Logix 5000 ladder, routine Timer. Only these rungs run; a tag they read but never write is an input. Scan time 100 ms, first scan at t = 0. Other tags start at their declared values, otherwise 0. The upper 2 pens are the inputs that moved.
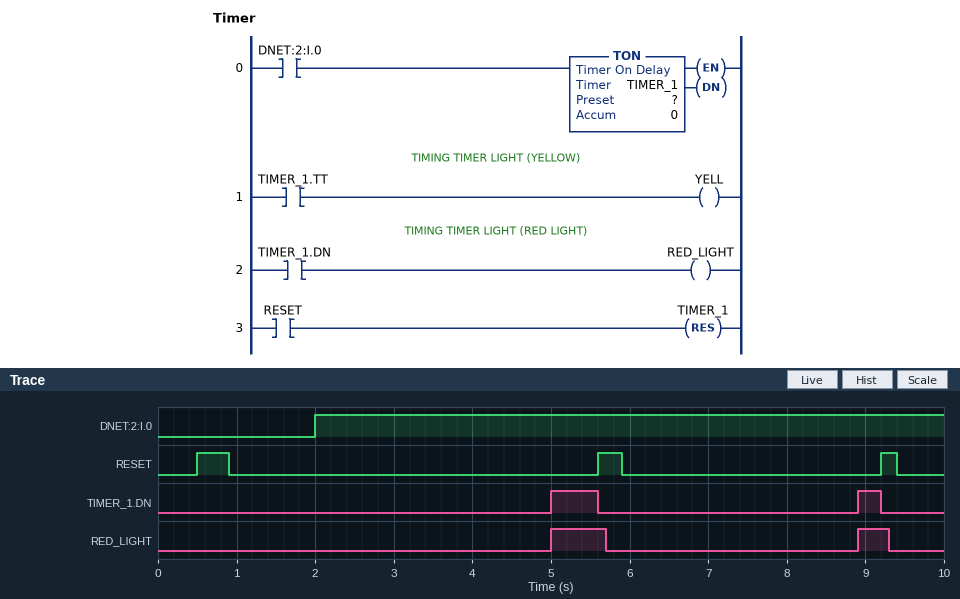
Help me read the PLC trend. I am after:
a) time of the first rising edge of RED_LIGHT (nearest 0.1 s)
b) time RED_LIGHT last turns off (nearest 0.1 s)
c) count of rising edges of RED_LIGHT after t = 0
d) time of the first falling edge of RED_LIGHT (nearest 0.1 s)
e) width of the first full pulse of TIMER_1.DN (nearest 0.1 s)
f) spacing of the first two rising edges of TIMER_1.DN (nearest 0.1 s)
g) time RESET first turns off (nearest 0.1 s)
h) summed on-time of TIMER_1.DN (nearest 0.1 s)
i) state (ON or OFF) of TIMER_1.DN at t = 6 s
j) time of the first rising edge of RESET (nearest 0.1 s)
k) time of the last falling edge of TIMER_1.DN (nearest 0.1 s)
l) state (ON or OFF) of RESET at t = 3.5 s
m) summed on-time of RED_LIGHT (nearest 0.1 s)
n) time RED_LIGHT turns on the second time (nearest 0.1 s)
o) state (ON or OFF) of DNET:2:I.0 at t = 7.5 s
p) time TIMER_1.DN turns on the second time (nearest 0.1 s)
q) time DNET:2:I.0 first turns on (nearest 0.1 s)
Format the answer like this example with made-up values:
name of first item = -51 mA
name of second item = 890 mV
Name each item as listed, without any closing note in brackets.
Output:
time of the first rising edge of RED_LIGHT = 5.0 s
time RED_LIGHT last turns off = 9.3 s
count of rising edges of RED_LIGHT after t = 0 = 2
time of the first falling edge of RED_LIGHT = 5.7 s
width of the first full pulse of TIMER_1.DN = 0.6 s
spacing of the first two rising edges of TIMER_1.DN = 3.9 s
time RESET first turns off = 0.9 s
summed on-time of TIMER_1.DN = 0.9 s
state (ON or OFF) of TIMER_1.DN at t = 6 s = OFF
time of the first rising edge of RESET = 0.5 s
time of the last falling edge of TIMER_1.DN = 9.2 s
state (ON or OFF) of RESET at t = 3.5 s = OFF
summed on-time of RED_LIGHT = 1.1 s
time RED_LIGHT turns on the second time = 8.9 s
state (ON or OFF) of DNET:2:I.0 at t = 7.5 s = ON
time TIMER_1.DN turns on the second time = 8.9 s
time DNET:2:I.0 first turns on = 2.0 s
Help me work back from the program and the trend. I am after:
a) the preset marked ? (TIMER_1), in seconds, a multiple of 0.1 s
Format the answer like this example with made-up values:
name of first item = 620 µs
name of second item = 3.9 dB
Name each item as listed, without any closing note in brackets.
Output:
the preset marked ? (TIMER_1), in seconds, a multiple of 0.1 s = 3.0 s
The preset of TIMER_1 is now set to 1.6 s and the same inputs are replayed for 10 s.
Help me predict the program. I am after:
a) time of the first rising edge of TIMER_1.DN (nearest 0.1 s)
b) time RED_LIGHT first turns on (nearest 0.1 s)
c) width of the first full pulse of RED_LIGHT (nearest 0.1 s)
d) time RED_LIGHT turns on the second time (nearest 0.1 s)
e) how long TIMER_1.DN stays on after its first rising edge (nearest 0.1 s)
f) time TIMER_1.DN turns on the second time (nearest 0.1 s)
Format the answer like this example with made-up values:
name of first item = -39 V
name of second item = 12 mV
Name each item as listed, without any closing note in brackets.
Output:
time of the first rising edge of TIMER_1.DN = 3.6 s
time RED_LIGHT first turns on = 3.6 s
width of the first full pulse of RED_LIGHT = 2.1 s
time RED_LIGHT turns on the second time = 7.5 s
how long TIMER_1.DN stays on after its first rising edge = 2.0 s
time TIMER_1.DN turns on the second time = 7.5 s
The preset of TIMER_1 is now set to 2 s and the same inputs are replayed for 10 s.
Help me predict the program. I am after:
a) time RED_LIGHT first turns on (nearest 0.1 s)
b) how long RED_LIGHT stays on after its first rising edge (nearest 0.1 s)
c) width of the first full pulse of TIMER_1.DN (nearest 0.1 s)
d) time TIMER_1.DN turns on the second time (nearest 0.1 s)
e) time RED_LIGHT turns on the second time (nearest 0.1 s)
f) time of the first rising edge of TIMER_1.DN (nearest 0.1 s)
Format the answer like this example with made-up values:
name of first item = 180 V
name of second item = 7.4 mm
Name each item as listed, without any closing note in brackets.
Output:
time RED_LIGHT first turns on = 4.0 s
how long RED_LIGHT stays on after its first rising edge = 1.7 s
width of the first full pulse of TIMER_1.DN = 1.6 s
time TIMER_1.DN turns on the second time = 7.9 s
time RED_LIGHT turns on the second time = 7.9 s
time of the first rising edge of TIMER_1.DN = 4.0 s
